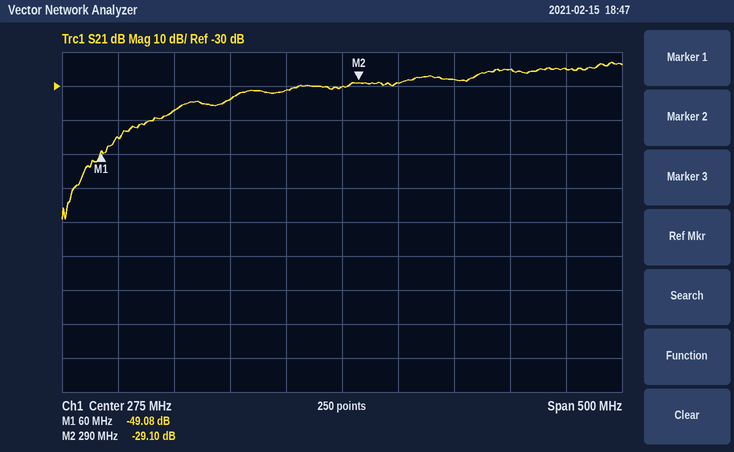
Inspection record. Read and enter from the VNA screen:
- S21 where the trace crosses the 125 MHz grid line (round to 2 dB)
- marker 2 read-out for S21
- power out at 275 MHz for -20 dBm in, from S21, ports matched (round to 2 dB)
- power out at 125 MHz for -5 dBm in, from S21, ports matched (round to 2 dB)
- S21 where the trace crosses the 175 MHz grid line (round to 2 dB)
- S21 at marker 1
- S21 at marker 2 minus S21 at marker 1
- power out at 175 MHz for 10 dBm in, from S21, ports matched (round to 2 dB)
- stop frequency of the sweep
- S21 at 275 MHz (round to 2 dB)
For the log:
-38 dB
-29.10 dB
-50 dBm
-42 dBm
-34 dB
-49.08 dB
19.98 dB
-24 dBm
525 MHz
-30 dB
